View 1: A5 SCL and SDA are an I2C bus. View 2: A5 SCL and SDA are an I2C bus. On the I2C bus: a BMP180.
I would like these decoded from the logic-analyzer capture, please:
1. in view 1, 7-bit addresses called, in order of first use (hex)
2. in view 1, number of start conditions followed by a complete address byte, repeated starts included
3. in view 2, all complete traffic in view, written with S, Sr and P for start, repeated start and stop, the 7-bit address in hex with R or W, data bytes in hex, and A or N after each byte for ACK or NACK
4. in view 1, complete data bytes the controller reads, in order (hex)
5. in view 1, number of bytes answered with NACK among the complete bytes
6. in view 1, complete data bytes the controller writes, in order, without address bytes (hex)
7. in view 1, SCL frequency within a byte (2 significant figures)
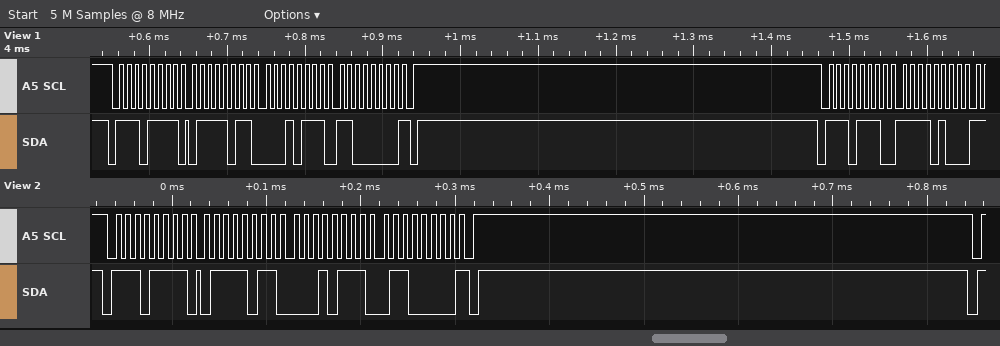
0x77
2
S 77R A 7B A 17 A 60 N P
7B 17 C0
1
F4
100 kHz
